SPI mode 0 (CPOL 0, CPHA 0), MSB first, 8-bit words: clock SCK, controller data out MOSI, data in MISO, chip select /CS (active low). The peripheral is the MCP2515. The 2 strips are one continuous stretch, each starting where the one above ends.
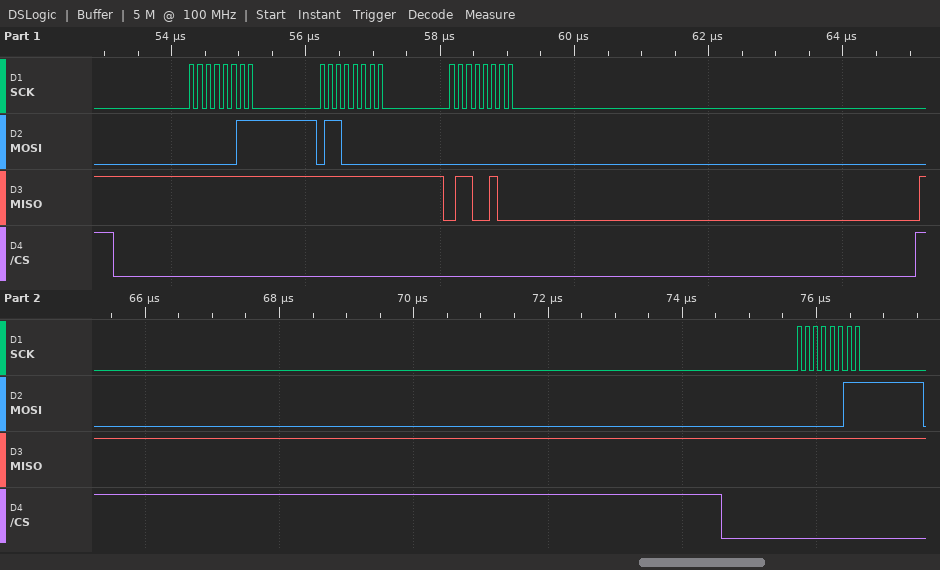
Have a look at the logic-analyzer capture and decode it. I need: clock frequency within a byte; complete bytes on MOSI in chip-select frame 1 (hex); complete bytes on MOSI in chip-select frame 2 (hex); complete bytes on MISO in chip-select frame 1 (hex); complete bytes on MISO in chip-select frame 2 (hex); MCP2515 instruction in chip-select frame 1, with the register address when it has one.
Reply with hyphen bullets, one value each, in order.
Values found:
- 8 MHz
- 03 60 00
- 03
- FF FF 64
- FF
- READ 0x60
